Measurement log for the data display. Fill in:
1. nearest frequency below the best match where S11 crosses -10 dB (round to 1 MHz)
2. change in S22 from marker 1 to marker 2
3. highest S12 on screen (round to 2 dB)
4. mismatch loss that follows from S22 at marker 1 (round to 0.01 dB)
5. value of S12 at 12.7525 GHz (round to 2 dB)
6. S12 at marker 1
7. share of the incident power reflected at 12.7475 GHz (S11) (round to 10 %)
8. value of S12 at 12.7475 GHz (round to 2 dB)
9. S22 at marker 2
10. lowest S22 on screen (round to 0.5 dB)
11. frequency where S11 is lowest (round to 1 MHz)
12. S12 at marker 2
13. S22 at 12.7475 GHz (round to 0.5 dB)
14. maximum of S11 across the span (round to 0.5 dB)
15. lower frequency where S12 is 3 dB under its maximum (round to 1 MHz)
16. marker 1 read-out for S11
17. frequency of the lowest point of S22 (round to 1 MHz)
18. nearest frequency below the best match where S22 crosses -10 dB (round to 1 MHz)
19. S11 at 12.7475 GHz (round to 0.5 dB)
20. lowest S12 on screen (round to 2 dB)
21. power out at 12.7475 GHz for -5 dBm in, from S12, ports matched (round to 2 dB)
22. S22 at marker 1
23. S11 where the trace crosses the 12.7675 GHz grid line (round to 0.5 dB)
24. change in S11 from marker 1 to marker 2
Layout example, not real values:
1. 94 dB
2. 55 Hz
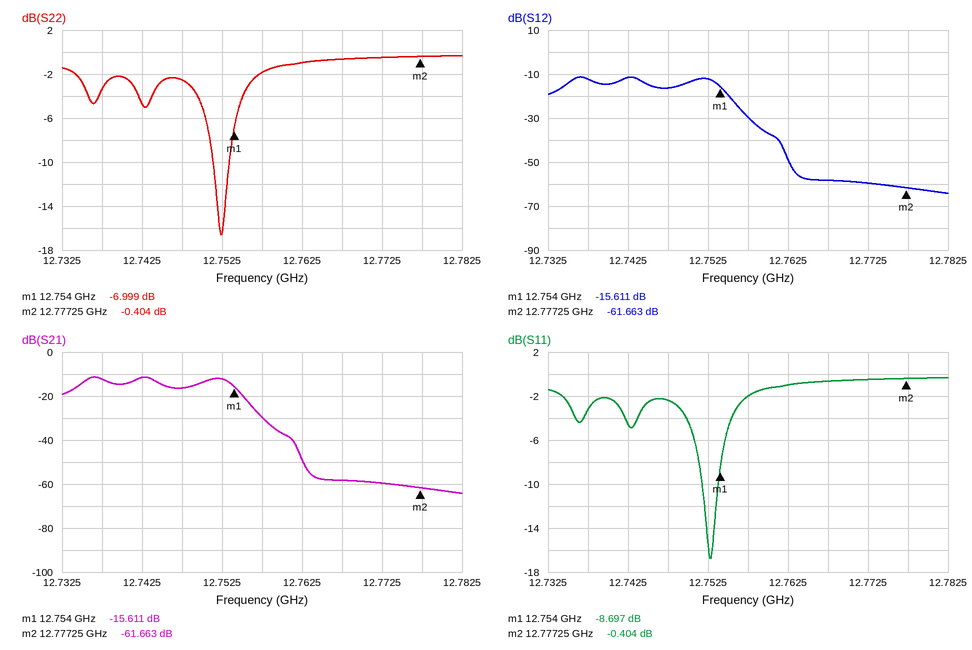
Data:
1. 12.752 GHz
2. 6.595 dB
3. -12 dB
4. 0.97 dB
5. -12 dB
6. -15.611 dB
7. 60 %
8. -16 dB
9. -0.404 dB
10. -16.5 dB
11. 12.753 GHz
12. -61.663 dB
13. -2.5 dB
14. -0.5 dB
15. 12.735 GHz
16. -8.697 dB
17. 12.752 GHz
18. 12.751 GHz
19. -2.5 dB
20. -64 dB
21. -22 dBm
22. -6.999 dB
23. -0.5 dB
24. 8.293 dB
